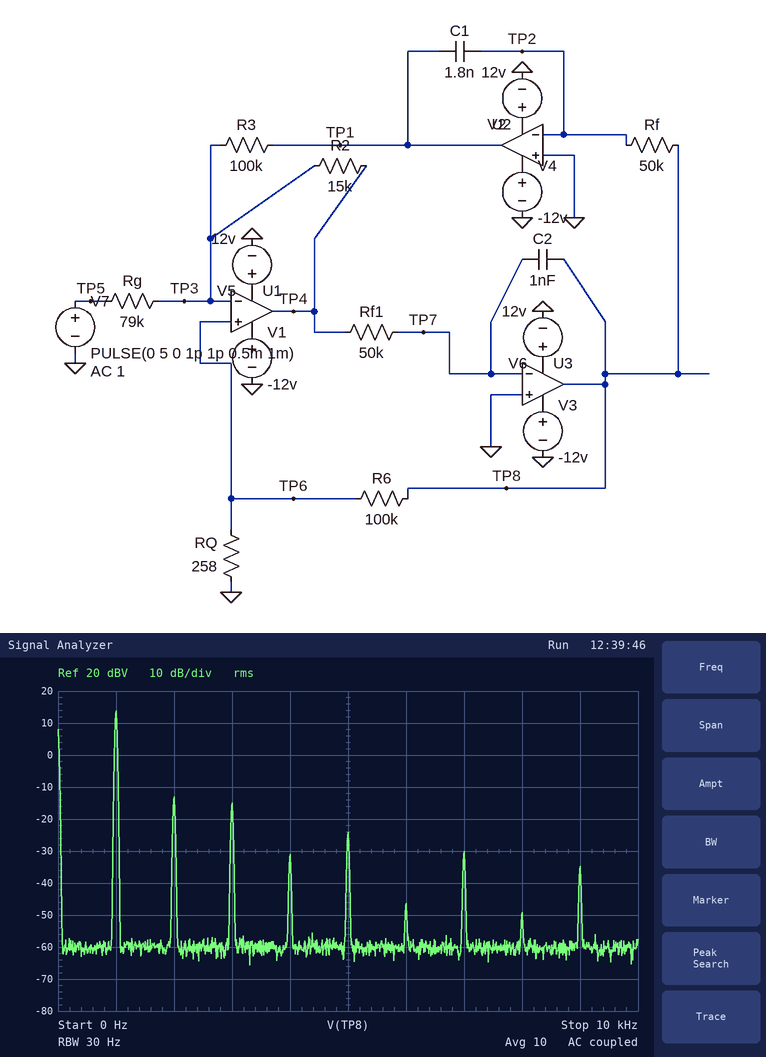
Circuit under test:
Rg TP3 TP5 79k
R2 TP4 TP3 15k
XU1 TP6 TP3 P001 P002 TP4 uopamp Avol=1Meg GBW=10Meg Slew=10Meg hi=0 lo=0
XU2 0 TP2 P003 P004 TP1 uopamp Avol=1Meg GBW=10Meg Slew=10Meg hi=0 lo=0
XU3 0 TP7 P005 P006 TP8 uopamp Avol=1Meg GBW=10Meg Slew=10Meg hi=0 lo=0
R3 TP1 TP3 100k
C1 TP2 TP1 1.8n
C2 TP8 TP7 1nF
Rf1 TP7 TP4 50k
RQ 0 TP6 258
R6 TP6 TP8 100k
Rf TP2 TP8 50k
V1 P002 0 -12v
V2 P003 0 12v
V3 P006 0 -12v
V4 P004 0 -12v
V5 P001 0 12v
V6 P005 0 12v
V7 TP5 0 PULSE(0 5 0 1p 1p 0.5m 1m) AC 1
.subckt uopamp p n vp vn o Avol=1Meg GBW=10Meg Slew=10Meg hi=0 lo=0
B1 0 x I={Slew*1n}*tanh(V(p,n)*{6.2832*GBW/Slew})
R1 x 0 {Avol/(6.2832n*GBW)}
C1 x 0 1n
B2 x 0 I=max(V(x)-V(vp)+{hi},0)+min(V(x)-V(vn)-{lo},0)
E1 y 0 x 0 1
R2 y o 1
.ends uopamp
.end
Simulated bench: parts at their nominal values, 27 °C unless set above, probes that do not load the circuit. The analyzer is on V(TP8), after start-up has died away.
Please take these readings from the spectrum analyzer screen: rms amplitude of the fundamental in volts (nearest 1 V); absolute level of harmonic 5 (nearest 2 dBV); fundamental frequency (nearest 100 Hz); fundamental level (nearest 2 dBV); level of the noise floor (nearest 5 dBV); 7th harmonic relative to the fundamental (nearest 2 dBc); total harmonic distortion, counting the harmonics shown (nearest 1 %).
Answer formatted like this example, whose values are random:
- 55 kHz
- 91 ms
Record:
- 5 V
- -24 dBV
- 1.0 kHz
- 14 dBV
- -60 dBV
- -44 dBc
- 6 %
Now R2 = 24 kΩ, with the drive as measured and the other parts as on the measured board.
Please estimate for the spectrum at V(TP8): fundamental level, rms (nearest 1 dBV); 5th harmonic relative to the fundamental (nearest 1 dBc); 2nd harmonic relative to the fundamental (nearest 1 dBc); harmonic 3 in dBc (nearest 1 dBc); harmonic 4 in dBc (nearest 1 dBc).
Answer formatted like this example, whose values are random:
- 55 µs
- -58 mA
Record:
- 17 dBV
- -42 dBc
- -17 dBc
- -26 dBc
- -41 dBc
